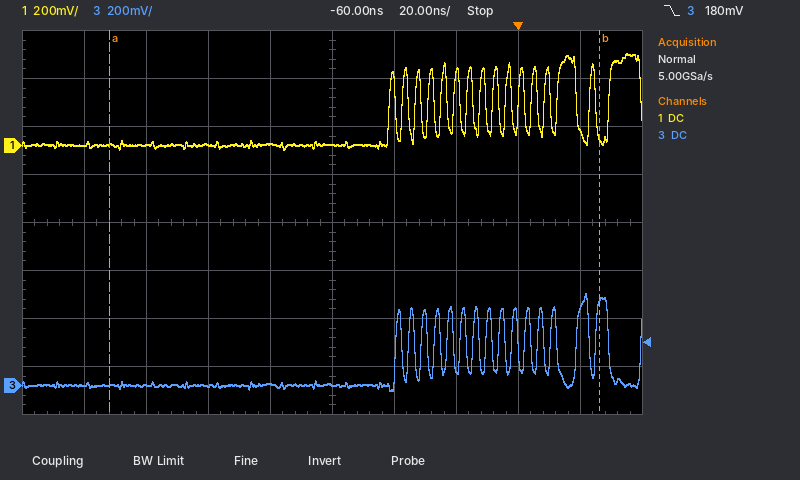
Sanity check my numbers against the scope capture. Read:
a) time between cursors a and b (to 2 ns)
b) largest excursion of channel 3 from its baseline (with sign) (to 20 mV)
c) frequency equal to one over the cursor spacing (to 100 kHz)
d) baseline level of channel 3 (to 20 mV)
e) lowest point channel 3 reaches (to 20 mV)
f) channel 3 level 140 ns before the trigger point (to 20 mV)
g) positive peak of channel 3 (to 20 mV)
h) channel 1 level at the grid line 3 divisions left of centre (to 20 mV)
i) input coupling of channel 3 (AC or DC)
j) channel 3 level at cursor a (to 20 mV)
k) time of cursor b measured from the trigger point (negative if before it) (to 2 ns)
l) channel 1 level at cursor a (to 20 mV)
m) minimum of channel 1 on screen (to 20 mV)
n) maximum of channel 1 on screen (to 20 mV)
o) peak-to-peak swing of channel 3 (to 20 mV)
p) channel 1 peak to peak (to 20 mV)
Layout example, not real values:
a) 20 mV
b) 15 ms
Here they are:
a) 158 ns
b) +380 mV
c) 6.3 MHz
d) 0 mV
e) -20 mV
f) 0 mV
g) 380 mV
h) 0 mV
i) DC
j) 0 mV
k) +26 ns
l) 0 mV
m) -20 mV
n) 380 mV
o) 400 mV
p) 400 mV
